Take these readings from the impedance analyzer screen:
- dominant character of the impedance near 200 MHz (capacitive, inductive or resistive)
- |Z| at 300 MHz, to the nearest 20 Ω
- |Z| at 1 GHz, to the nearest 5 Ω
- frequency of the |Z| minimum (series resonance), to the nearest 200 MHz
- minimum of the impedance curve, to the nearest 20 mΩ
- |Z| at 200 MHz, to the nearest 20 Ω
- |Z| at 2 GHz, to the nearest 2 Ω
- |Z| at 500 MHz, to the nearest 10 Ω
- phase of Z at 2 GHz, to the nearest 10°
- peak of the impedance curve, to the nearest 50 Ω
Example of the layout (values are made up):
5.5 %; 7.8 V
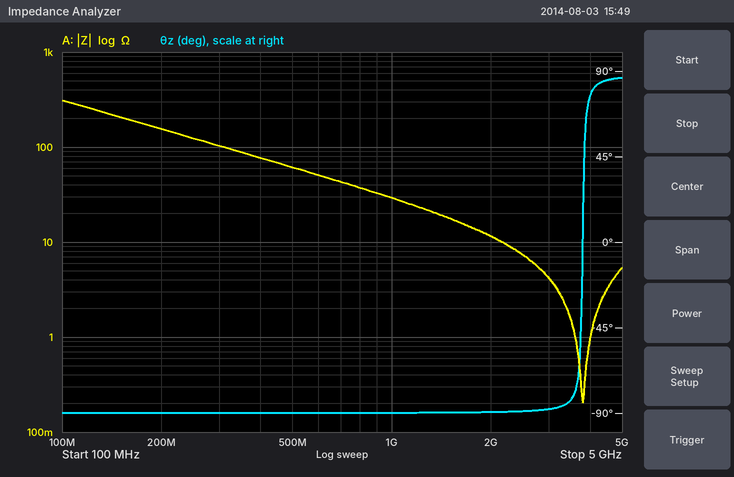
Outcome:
capacitive; 100 Ω; 30 Ω; 3.8 GHz; 200 mΩ; 160 Ω; 12 Ω; 60 Ω; -90°; 300 Ω
